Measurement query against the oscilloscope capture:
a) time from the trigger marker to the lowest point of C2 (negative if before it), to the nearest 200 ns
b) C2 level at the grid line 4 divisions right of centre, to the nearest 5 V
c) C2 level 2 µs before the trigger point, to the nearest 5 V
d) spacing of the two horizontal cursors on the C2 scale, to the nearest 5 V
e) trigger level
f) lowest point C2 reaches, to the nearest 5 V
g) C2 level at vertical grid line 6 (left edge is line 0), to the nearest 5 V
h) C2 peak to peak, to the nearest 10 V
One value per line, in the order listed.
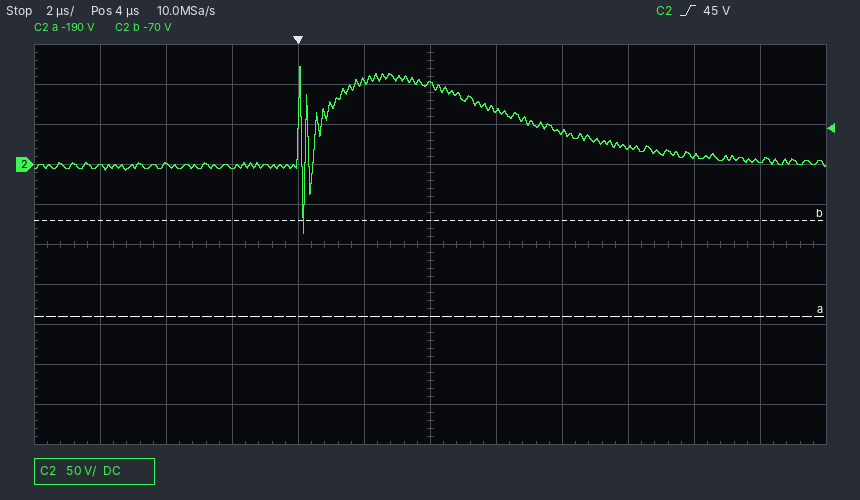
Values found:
+200 ns
10 V
-5 V
120 V
45 V
-85 V
100 V
210 V
